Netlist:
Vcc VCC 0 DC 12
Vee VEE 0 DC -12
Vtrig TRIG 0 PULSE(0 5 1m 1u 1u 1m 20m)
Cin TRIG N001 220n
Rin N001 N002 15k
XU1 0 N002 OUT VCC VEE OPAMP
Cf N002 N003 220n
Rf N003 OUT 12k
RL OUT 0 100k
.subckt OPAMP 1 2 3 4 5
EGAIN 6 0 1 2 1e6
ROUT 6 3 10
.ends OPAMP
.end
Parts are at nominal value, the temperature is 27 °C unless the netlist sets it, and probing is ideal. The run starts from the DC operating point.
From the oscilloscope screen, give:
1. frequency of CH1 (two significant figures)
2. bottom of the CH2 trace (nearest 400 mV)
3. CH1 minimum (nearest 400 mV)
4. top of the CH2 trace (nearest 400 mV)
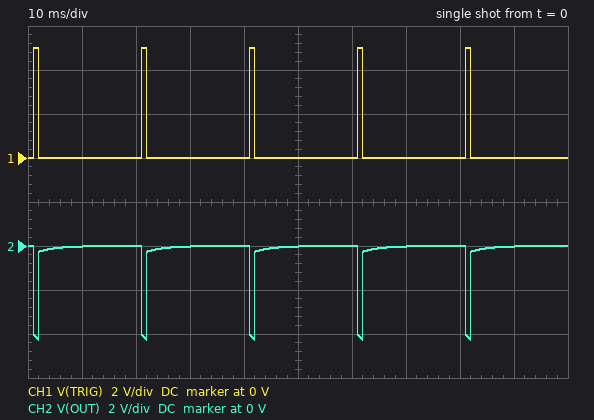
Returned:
50 Hz
-4.4 V
0 V
0 V
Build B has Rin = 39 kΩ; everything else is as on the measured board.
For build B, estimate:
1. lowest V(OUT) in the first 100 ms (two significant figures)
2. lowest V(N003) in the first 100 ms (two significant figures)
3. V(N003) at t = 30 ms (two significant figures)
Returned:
-2.0 V
-610 mV
-240 mV
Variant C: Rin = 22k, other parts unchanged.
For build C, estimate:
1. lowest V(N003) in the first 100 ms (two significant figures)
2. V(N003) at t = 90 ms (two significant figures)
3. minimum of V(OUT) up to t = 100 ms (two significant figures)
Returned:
-950 mV
-180 mV
-3.2 V
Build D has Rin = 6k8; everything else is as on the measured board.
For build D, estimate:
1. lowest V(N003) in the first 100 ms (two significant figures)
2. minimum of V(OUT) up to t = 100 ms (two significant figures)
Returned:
-2.4 V
-8.8 V
